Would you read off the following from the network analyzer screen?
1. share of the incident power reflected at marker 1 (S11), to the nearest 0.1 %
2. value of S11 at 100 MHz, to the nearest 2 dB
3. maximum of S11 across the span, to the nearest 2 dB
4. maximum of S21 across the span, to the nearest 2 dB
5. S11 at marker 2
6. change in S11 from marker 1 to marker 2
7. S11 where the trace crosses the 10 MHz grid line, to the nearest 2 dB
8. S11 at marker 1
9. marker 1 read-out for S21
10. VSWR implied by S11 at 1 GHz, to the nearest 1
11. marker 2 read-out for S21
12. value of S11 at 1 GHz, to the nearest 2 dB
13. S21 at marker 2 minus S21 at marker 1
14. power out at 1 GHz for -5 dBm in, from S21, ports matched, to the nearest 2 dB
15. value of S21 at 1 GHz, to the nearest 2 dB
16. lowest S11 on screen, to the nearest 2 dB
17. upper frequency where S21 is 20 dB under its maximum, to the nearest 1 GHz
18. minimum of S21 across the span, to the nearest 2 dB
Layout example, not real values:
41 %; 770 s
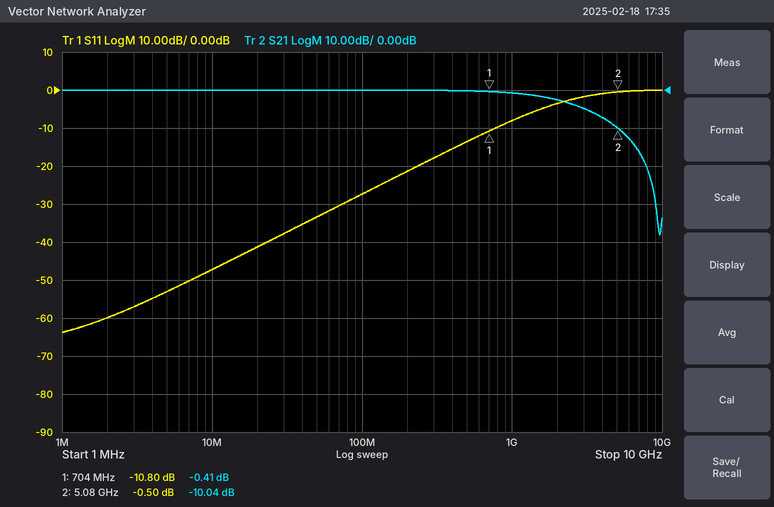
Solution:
8.3 %; -28 dB; 0 dB; 0 dB; -0.50 dB; 10.30 dB; -48 dB; -10.80 dB; -0.41 dB; 2; -10.04 dB; -8 dB; -9.63 dB; -6 dBm; 0 dB; -64 dB; 8 GHz; -38 dB
